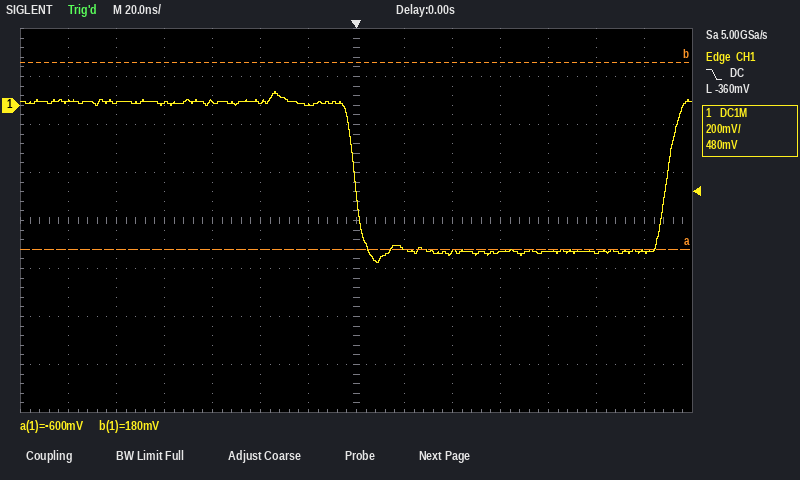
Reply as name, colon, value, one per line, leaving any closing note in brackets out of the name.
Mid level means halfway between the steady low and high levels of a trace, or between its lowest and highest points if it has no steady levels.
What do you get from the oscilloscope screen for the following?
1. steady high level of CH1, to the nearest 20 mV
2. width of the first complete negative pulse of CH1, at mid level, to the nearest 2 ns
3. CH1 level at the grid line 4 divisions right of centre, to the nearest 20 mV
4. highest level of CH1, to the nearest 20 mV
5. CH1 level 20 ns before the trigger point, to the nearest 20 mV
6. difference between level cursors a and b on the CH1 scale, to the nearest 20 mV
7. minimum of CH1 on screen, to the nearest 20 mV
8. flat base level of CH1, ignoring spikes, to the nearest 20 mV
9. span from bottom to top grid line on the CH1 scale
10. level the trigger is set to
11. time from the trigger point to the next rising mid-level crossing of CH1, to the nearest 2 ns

steady high level of CH1, to the nearest 20 mV: 20 mV
width of the first complete negative pulse of CH1, at mid level, to the nearest 2 ns: 130 ns
CH1 level at the grid line 4 divisions right of centre, to the nearest 20 mV: -600 mV
highest level of CH1, to the nearest 20 mV: 60 mV
CH1 level 20 ns before the trigger point, to the nearest 20 mV: 0 mV
difference between level cursors a and b on the CH1 scale, to the nearest 20 mV: 780 mV
minimum of CH1 on screen, to the nearest 20 mV: -660 mV
flat base level of CH1, ignoring spikes, to the nearest 20 mV: -600 mV
span from bottom to top grid line on the CH1 scale: 1.6 V
level the trigger is set to: -360 mV
time from the trigger point to the next rising mid-level crossing of CH1, to the nearest 2 ns: 130 ns
